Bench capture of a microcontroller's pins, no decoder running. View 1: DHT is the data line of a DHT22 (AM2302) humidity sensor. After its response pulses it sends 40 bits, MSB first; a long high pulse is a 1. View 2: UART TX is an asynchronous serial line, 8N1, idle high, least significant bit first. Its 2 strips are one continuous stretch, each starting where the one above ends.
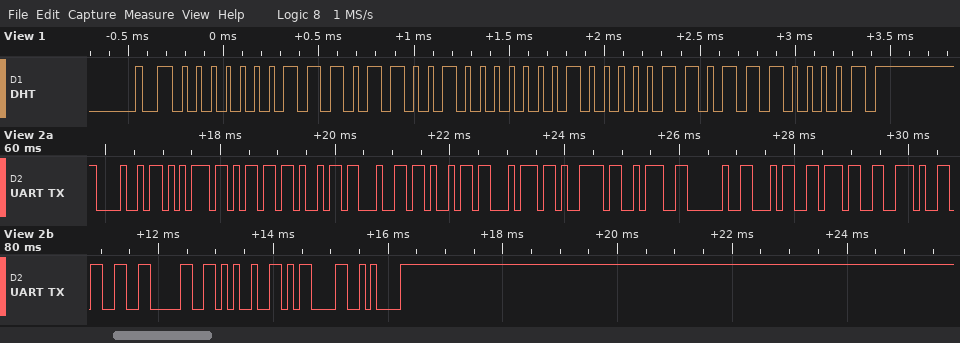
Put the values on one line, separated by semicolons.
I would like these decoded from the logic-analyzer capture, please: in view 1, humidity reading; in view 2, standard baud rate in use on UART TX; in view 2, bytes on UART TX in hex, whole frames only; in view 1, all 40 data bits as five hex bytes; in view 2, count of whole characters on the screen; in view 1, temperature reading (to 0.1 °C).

47.3 %; 9600 baud; 48 75 6D 69 64 69 74 79 3A 20 34 37 2E 33 30 25 0D 0A; 01 D9 01 06 E1; 18; 26.2 °C
